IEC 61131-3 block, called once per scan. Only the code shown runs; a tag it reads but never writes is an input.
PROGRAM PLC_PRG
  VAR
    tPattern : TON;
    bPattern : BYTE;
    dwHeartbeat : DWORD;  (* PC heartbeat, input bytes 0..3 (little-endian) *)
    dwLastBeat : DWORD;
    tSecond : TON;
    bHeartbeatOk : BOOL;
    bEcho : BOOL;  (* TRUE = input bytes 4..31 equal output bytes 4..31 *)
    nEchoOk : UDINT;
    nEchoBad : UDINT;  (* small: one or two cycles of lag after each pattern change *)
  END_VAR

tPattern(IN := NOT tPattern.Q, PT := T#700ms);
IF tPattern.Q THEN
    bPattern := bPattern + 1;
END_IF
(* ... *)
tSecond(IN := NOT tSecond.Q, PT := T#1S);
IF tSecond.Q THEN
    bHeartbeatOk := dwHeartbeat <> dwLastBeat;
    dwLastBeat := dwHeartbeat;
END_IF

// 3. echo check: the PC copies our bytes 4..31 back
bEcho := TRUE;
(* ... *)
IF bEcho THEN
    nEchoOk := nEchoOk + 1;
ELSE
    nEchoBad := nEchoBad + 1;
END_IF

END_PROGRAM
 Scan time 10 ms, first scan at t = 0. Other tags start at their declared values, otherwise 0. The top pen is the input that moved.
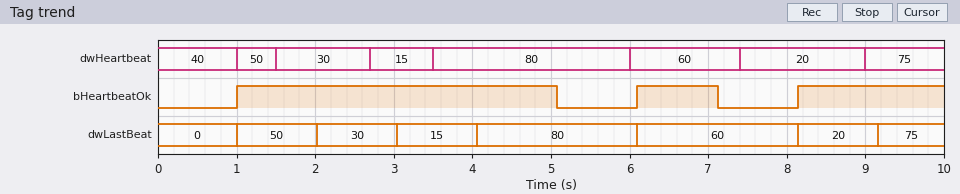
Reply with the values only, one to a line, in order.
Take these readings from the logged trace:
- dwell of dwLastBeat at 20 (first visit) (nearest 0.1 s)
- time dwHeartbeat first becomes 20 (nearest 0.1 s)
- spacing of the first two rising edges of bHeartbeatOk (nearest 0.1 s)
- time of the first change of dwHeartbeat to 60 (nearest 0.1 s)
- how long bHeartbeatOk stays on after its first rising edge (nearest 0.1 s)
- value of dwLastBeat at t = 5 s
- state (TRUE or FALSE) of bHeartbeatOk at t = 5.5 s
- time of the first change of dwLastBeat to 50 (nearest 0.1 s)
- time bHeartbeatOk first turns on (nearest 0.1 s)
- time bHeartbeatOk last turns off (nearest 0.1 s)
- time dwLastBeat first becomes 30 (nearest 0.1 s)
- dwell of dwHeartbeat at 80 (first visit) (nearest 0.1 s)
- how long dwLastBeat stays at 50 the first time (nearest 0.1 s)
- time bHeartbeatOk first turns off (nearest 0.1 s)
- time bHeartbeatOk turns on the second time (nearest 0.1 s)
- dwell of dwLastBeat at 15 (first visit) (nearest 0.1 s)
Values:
1.0 s
7.4 s
5.1 s
6.0 s
4.1 s
80
FALSE
1.0 s
1.0 s
7.1 s
2.0 s
2.5 s
1.0 s
5.1 s
6.1 s
1.0 s
